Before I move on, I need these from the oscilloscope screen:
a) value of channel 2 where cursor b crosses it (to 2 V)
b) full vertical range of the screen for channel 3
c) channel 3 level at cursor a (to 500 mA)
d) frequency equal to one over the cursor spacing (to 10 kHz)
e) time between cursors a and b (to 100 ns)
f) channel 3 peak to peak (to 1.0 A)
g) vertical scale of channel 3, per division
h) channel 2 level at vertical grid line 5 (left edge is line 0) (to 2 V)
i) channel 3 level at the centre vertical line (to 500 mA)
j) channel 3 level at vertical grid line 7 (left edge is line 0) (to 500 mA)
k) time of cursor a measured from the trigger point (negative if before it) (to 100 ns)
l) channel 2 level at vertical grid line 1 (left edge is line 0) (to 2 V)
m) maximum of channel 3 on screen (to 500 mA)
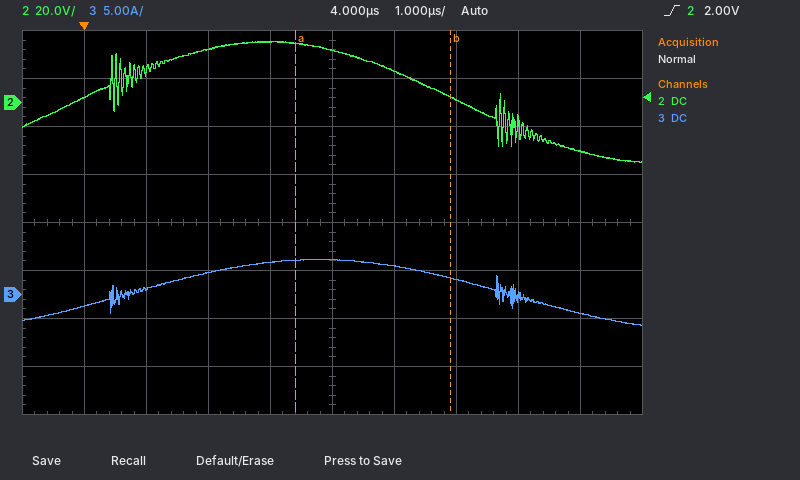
2 V
40 A
3.5 A
400 kHz
2.5 µs
7.0 A
5 A
22 V
3.5 A
1.5 A
+3.4 µs
2 V
3.5 A
